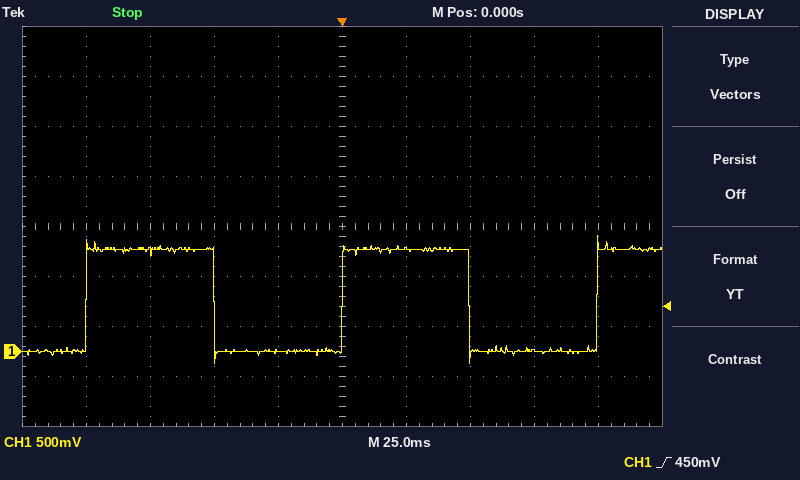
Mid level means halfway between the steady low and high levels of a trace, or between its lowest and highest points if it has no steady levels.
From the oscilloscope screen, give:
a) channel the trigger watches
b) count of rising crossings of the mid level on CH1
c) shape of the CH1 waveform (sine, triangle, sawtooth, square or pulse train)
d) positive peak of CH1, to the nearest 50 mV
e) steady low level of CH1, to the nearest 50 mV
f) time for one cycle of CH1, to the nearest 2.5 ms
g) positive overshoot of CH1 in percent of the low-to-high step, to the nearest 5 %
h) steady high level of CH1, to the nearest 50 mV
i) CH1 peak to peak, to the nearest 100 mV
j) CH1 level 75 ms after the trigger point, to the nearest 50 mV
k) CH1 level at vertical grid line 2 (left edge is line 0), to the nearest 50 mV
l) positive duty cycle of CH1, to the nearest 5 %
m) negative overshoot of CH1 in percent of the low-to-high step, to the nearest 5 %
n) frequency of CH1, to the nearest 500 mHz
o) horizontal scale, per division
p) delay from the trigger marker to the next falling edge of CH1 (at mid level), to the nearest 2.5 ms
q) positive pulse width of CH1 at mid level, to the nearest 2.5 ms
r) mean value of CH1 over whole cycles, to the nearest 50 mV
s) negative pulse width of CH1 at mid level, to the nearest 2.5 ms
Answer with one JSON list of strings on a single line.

["CH1", "3", "square", "1.15 V", "0 mV", "100.0 ms", "15 %", "1.00 V", "1.30 V", "0 mV", "1.00 V", "50 %", "10 %", "10.0 Hz", "25 ms", "50.0 ms", "50.0 ms", "500 mV", "50.0 ms"]
